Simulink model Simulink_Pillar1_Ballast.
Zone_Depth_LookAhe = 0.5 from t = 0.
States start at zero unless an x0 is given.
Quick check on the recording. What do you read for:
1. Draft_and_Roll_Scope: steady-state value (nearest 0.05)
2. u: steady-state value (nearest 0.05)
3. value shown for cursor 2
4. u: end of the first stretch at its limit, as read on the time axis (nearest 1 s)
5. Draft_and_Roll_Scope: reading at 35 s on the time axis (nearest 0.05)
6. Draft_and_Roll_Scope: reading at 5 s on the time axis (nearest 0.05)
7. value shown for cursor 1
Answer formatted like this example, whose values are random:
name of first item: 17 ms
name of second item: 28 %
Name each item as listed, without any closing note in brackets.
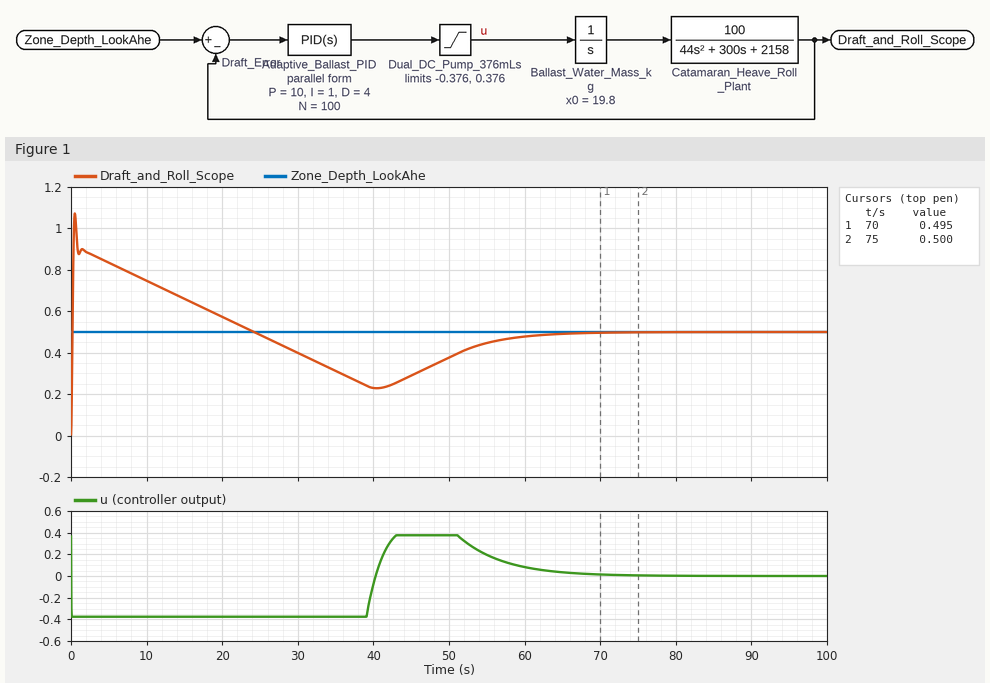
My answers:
Draft_and_Roll_Scope: steady-state value: 0.50
u: steady-state value: 0.00
value shown for cursor 2: 0.500
u: end of the first stretch at its limit, as read on the time axis: 39 s
Draft_and_Roll_Scope: reading at 35 s on the time axis: 0.30
Draft_and_Roll_Scope: reading at 5 s on the time axis: 0.85
value shown for cursor 1: 0.495
